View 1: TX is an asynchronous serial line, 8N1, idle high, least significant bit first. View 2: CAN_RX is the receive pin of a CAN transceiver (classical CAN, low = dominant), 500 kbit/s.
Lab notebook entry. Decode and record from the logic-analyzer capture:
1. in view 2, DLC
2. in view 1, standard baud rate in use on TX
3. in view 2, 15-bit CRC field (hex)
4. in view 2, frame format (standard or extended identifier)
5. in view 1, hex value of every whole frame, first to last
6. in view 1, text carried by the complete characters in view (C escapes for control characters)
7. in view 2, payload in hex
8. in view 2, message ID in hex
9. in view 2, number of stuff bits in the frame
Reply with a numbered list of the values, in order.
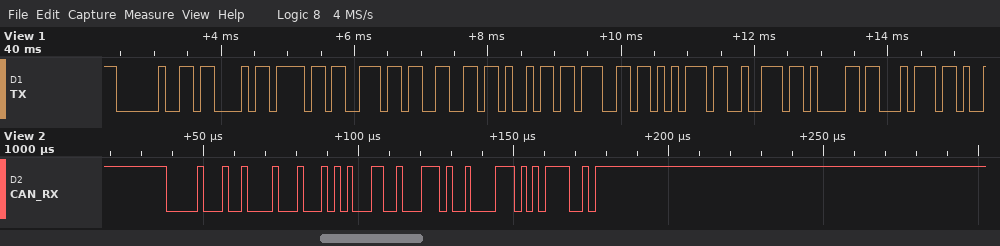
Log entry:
1. 4
2. 9600 baud
3. 0x3ABC
4. standard
5. 20 43 6F 6E 66 69 67 75 72 61 74
6. " Configurat"
7. 45 46 47 48
8. 0x009
9. 1
